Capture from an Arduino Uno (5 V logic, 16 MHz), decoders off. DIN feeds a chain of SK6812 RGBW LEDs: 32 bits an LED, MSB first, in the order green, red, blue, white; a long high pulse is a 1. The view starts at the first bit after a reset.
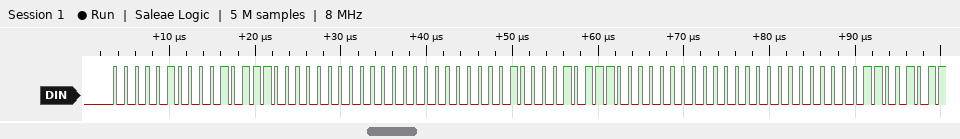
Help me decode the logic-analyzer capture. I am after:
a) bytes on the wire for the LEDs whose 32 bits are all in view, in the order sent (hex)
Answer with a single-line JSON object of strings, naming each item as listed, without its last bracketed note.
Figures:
{"bytes on the wire for the LEDs whose 32 bits are all in view, in the order sent": "04 2E 00 00 04 2E 00 00"}
